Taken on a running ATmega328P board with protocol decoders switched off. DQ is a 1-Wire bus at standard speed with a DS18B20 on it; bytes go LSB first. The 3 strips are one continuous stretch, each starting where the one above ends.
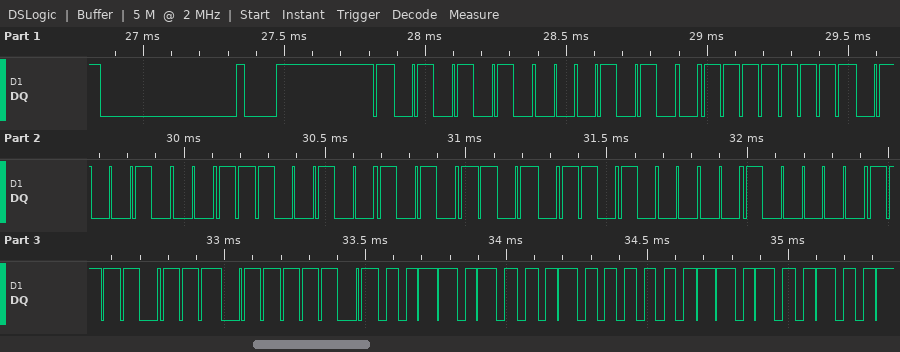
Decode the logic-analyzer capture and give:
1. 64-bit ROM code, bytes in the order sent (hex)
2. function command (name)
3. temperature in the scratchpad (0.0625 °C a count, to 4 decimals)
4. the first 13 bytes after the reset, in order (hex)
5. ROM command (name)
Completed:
28 FF 12 27 B5 16 04 EF
Read Scratchpad
34.7500 °C
55 28 FF 12 27 B5 16 04 EF BE 2C 02 4B
Match ROM
